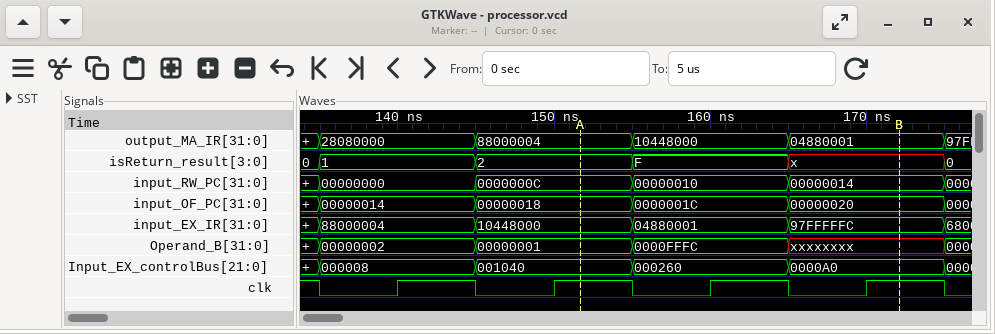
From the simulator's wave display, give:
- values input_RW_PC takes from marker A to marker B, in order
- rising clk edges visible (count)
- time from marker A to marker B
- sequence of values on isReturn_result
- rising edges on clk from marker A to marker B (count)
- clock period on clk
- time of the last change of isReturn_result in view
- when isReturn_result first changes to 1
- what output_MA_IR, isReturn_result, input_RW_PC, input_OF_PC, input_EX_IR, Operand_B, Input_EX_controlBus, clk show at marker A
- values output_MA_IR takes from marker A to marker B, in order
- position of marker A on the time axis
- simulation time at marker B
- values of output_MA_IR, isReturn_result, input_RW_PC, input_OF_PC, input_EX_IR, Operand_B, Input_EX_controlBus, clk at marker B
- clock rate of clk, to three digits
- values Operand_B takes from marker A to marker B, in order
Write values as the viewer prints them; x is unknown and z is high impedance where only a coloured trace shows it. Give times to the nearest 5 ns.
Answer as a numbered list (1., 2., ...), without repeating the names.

1. 0000000C, 00000010, 00000014
2. 4
3. 20 ns
4. 0, 1, 2, F, x, 0
5. 2
6. 10 ns
7. 175 ns
8. 135 ns
9. output_MA_IR=88000004, isReturn_result=2, input_RW_PC=0000000C, input_OF_PC=00000018, input_EX_IR=10448000, Operand_B=00000001, Input_EX_controlBus=001040, clk=1
10. 88000004, 10448000, 04880001
11. 150 ns
12. 170 ns
13. output_MA_IR=04880001, isReturn_result=x, input_RW_PC=00000014, input_OF_PC=00000020, input_EX_IR=97FFFFFC, Operand_B=xxxxxxxx, Input_EX_controlBus=0000A0, clk=1
14. 100 MHz
15. 00000001, 0000FFFC, xxxxxxxx
